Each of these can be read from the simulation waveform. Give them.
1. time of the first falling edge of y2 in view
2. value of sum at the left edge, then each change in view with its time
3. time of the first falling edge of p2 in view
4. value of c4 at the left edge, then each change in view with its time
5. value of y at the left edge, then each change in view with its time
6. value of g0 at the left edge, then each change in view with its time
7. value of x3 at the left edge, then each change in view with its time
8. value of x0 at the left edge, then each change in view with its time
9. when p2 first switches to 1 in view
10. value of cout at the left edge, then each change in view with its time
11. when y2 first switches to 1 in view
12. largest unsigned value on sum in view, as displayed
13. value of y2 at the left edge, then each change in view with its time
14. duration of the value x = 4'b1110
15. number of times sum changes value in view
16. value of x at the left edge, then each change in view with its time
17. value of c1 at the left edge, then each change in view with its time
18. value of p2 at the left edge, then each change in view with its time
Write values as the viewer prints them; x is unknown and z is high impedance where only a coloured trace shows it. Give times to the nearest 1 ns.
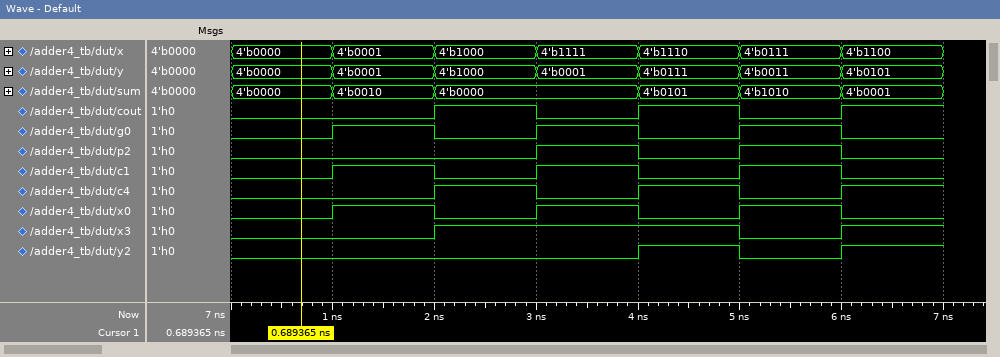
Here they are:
5 ns
4'b0000, 4'b0010 at 1 ns, 4'b0000 at 2 ns, 4'b0101 at 4 ns, 4'b1010 at 5 ns, 4'b0001 at 6 ns
4 ns
0, 1 at 2 ns, 0 at 3 ns, 1 at 4 ns, 0 at 5 ns, 1 at 6 ns
4'b0000, 4'b0001 at 1 ns, 4'b1000 at 2 ns, 4'b0001 at 3 ns, 4'b0111 at 4 ns, 4'b0011 at 5 ns, 4'b0101 at 6 ns
0, 1 at 1 ns, 0 at 2 ns, 1 at 3 ns, 0 at 4 ns, 1 at 5 ns, 0 at 6 ns
0, 1 at 2 ns, 0 at 5 ns, 1 at 6 ns
0, 1 at 1 ns, 0 at 2 ns, 1 at 3 ns, 0 at 4 ns, 1 at 5 ns, 0 at 6 ns
3 ns
0, 1 at 2 ns, 0 at 3 ns, 1 at 4 ns, 0 at 5 ns, 1 at 6 ns
4 ns
4'b1010
0, 1 at 4 ns, 0 at 5 ns, 1 at 6 ns
1 ns
5
4'b0000, 4'b0001 at 1 ns, 4'b1000 at 2 ns, 4'b1111 at 3 ns, 4'b1110 at 4 ns, 4'b0111 at 5 ns, 4'b1100 at 6 ns
0, 1 at 1 ns, 0 at 2 ns, 1 at 3 ns, 0 at 4 ns, 1 at 5 ns, 0 at 6 ns
0, 1 at 3 ns, 0 at 4 ns, 1 at 5 ns, 0 at 6 ns
